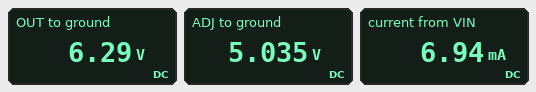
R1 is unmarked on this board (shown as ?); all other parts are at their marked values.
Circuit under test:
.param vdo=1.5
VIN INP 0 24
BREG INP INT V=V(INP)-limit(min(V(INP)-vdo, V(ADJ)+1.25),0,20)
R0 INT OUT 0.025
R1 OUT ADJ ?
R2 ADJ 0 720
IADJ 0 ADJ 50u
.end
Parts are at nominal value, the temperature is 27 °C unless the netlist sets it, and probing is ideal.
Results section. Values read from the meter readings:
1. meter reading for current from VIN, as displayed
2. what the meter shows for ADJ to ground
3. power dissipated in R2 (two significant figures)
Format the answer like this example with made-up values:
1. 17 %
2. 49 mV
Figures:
1. 6.94 mA
2. 5.035 V
3. 35 mW
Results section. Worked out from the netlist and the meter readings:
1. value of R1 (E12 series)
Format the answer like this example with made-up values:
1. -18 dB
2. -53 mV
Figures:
1. 180 Ω
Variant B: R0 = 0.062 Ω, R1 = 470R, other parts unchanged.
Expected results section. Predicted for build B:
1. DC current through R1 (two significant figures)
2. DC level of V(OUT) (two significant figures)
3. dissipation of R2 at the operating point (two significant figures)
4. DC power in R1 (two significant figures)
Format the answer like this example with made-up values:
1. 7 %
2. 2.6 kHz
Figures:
1. 2.7 mA
2. 3.2 V
3. 5.3 mW
4. 3.3 mW
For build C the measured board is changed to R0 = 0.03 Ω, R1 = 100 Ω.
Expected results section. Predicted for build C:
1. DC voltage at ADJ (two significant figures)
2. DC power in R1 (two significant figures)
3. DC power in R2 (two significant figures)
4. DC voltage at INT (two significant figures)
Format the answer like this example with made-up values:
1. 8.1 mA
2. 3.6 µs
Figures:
1. 9.0 V
2. 16 mW
3. 110 mW
4. 10 V
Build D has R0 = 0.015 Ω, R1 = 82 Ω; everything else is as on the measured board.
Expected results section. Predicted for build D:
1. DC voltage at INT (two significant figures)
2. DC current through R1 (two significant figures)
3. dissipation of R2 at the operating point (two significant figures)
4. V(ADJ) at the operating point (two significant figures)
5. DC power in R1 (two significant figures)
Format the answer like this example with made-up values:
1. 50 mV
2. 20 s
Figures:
1. 12 V
2. 15 mA
3. 170 mW
4. 11 V
5. 19 mW
